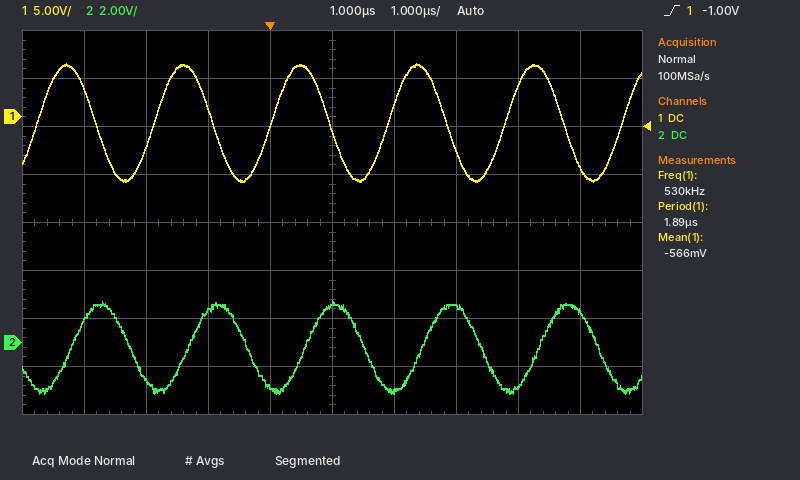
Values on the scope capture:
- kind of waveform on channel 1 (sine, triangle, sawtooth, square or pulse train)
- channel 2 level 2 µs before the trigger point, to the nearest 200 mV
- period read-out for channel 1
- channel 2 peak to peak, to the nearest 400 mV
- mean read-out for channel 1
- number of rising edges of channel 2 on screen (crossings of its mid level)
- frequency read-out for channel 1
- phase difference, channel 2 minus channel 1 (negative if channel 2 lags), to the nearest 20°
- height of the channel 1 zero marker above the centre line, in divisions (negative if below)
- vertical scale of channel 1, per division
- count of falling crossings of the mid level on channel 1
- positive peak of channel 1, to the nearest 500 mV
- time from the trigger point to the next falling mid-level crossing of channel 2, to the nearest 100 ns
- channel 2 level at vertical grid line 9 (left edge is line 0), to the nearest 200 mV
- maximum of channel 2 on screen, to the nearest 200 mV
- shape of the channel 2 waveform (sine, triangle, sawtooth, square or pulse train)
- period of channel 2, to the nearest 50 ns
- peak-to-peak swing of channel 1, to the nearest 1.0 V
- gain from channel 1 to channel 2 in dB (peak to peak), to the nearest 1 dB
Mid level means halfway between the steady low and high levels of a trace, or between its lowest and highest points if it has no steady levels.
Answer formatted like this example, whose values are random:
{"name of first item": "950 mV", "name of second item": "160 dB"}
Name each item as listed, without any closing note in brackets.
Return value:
{"kind of waveform on channel 1": "sine", "channel 2 level 2 µs before the trigger point, to the nearest 200 mV": "-1.6 V", "period read-out for channel 1": "1.89 µs", "channel 2 peak to peak, to the nearest 400 mV": "4.0 V", "mean read-out for channel 1": "-566 mV", "number of rising edges of channel 2 on screen": "5", "frequency read-out for channel 1": "530 kHz", "phase difference, channel 2 minus channel 1 (negative if channel 2 lags), to the nearest 20°": "-100°", "height of the channel 1 zero marker above the centre line, in divisions": "+2.2 div", "vertical scale of channel 1, per division": "5 V", "count of falling crossings of the mid level on channel 1": "5", "positive peak of channel 1, to the nearest 500 mV": "5.5 V", "time from the trigger point to the next falling mid-level crossing of channel 2, to the nearest 100 ns": "1.5 µs", "channel 2 level at vertical grid line 9 (left edge is line 0), to the nearest 200 mV": "1.2 V", "maximum of channel 2 on screen, to the nearest 200 mV": "1.8 V", "shape of the channel 2 waveform": "sine", "period of channel 2, to the nearest 50 ns": "1.90 µs", "peak-to-peak swing of channel 1, to the nearest 1.0 V": "12.0 V", "gain from channel 1 to channel 2 in dB (peak to peak), to the nearest 1 dB": "-10 dB"}
